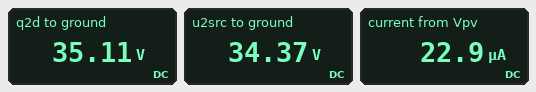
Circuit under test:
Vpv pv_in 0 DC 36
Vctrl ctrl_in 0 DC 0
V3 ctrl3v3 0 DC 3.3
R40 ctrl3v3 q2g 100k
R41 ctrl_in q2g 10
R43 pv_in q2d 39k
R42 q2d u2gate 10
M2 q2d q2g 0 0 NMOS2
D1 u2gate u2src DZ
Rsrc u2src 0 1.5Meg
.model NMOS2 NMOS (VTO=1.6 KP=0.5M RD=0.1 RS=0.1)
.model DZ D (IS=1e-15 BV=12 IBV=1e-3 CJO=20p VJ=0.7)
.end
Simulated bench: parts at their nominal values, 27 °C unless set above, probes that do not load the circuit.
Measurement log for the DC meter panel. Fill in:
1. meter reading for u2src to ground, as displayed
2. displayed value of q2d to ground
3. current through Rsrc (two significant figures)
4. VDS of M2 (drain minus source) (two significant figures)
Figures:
34.37 V
35.11 V
23 µA
35 V
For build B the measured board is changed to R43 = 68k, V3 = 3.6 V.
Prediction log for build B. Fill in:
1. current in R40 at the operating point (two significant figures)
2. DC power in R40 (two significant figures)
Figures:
36 µA
130 µW
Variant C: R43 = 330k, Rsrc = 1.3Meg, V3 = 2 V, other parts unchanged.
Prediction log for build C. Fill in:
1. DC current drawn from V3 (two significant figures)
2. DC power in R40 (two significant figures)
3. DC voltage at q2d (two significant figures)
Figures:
20 µA
40 µW
29 V
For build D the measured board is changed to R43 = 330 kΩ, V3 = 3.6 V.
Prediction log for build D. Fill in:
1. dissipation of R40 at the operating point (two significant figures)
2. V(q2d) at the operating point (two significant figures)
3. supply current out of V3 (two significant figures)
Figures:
130 µW
30 V
36 µA
